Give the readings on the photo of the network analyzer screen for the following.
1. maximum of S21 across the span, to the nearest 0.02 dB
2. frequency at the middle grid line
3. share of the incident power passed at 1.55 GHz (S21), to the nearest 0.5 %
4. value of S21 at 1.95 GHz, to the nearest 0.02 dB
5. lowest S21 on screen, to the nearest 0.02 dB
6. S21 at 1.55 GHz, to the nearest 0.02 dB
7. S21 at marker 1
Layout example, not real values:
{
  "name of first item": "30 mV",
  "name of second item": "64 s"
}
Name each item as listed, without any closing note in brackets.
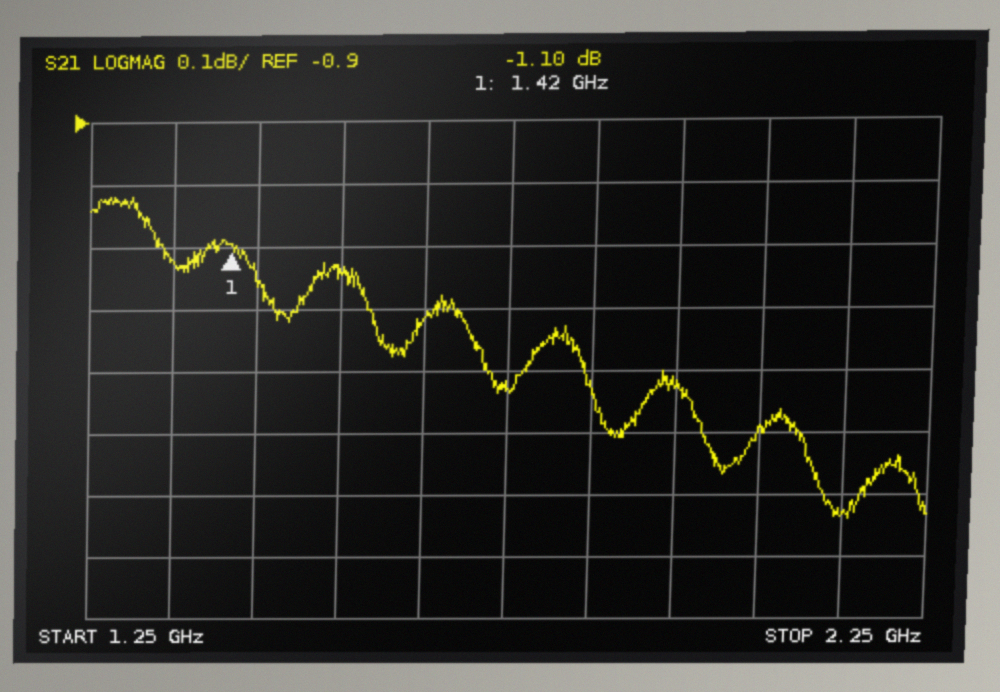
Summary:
{
  "maximum of S21 across the span, to the nearest 0.02 dB": "-1.02 dB",
  "frequency at the middle grid line": "1.75 GHz",
  "share of the incident power passed at 1.55 GHz (S21), to the nearest 0.5 %": "77.0 %",
  "value of S21 at 1.95 GHz, to the nearest 0.02 dB": "-1.32 dB",
  "lowest S21 on screen, to the nearest 0.02 dB": "-1.54 dB",
  "S21 at 1.55 GHz, to the nearest 0.02 dB": "-1.14 dB",
  "S21 at marker 1": "-1.10 dB"
}
